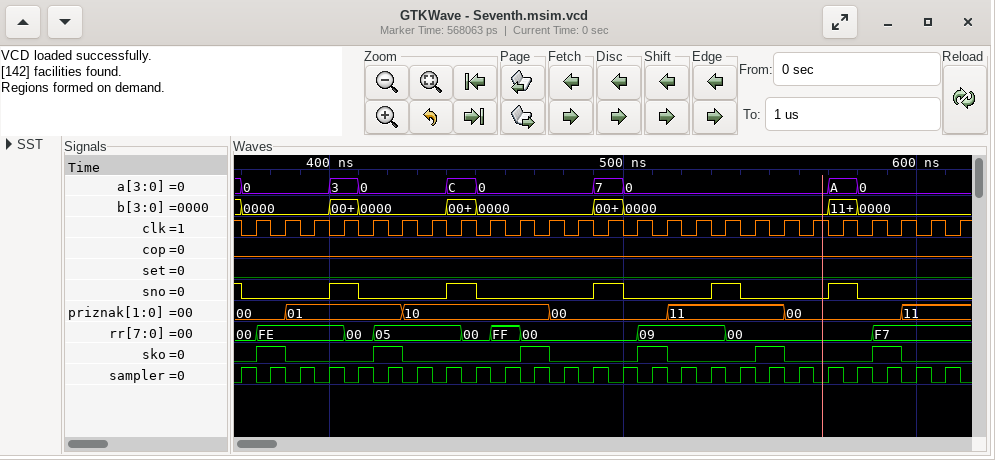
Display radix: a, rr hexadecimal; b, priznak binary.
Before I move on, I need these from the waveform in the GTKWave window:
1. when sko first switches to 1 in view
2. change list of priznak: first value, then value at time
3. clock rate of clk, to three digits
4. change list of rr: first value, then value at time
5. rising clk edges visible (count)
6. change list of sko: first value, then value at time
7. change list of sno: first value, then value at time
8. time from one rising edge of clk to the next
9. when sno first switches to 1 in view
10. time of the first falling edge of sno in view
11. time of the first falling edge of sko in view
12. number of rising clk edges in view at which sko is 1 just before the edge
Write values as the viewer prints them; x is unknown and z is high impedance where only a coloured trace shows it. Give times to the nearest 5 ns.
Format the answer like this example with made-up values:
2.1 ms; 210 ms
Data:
375 ns; 00, 01 at 385 ns, 10 at 425 ns, 00 at 475 ns, 11 at 515 ns, 00 at 555 ns, 11 at 595 ns; 100 MHz; 00, FE at 375 ns, 00 at 405 ns, 05 at 415 ns, 00 at 445 ns, FF at 455 ns, 00 at 465 ns, 09 at 505 ns, 00 at 535 ns, F7 at 585 ns; 25; 0, 1 at 375 ns, 0 at 385 ns, 1 at 415 ns, 0 at 425 ns, 1 at 465 ns, 0 at 475 ns, 1 at 505 ns, 0 at 515 ns, 1 at 545 ns, 0 at 555 ns, 1 at 585 ns, 0 at 595 ns; 1, 0 at 370 ns, 1 at 400 ns, 0 at 410 ns, 1 at 440 ns, 0 at 450 ns, 1 at 490 ns, 0 at 500 ns, 1 at 530 ns, 0 at 540 ns, 1 at 570 ns, 0 at 580 ns; 10 ns; 400 ns; 370 ns; 385 ns; 6
